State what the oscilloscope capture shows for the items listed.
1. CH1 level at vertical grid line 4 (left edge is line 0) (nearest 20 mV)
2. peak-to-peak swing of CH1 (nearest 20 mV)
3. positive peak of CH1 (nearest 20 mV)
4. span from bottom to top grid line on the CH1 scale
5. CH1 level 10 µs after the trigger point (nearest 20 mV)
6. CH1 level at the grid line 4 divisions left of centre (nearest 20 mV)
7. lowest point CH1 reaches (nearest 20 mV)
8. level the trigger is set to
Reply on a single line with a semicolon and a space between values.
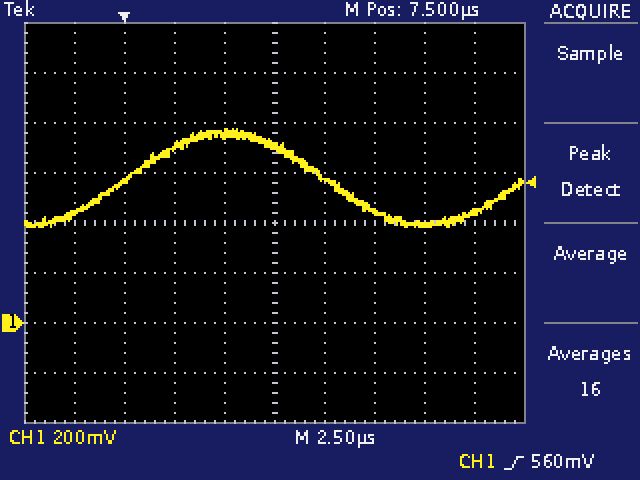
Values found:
760 mV; 400 mV; 780 mV; 1.6 V; 580 mV; 440 mV; 380 mV; 560 mV
